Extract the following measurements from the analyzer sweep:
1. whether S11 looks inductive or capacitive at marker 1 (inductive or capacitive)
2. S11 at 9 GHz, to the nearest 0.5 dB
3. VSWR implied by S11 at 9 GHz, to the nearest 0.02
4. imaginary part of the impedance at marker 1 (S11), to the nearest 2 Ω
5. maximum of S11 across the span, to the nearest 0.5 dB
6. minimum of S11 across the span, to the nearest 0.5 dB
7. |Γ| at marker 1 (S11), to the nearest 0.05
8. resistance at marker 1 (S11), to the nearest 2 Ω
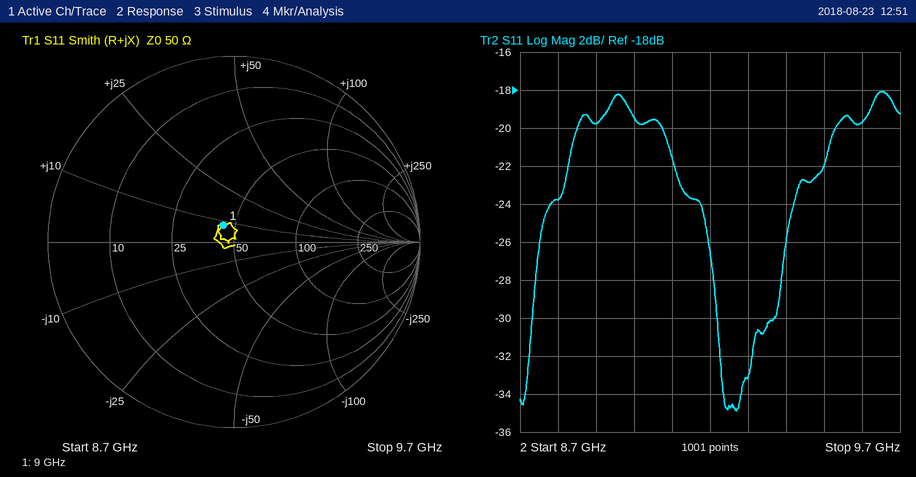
inductive
-19.5 dB
1.24
+8 Ω
-18.0 dB
-35.0 dB
0.10
44 Ω
